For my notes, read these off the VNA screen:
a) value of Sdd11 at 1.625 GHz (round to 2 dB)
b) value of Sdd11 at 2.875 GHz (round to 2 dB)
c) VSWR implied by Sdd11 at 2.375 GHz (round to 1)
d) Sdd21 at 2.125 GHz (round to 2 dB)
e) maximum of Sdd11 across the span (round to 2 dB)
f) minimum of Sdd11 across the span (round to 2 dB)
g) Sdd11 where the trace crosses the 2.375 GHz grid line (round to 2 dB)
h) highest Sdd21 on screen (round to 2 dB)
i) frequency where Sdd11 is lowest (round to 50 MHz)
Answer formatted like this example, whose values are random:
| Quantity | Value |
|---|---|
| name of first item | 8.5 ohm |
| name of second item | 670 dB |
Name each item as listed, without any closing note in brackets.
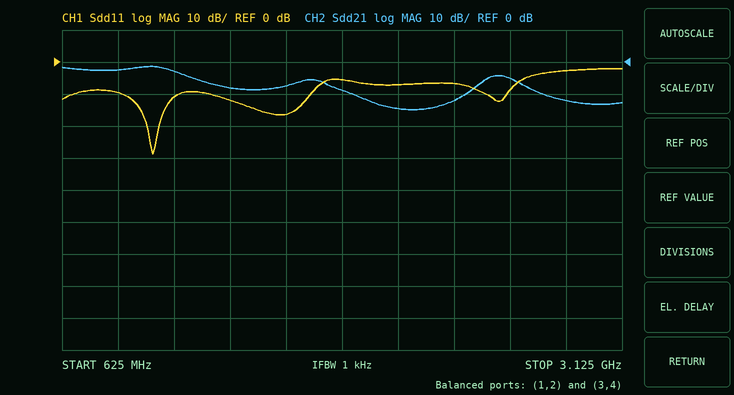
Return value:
| Quantity | Value |
|---|---|
| value of Sdd11 at 1.625 GHz | -16 dB |
| value of Sdd11 at 2.875 GHz | -2 dB |
| VSWR implied by Sdd11 at 2.375 GHz | 3 |
| Sdd21 at 2.125 GHz | -14 dB |
| maximum of Sdd11 across the span | -2 dB |
| minimum of Sdd11 across the span | -28 dB |
| Sdd11 where the trace crosses the 2.375 GHz grid line | -6 dB |
| highest Sdd21 on screen | -2 dB |
| frequency where Sdd11 is lowest | 1.05 GHz |
